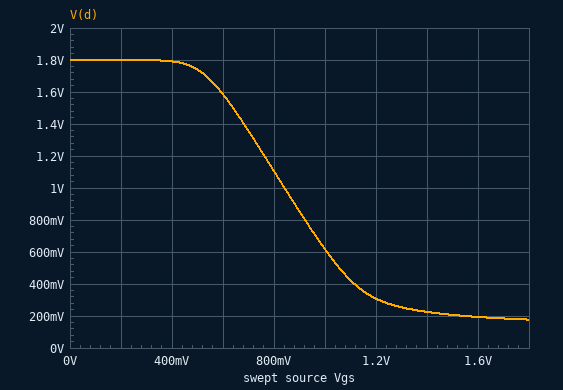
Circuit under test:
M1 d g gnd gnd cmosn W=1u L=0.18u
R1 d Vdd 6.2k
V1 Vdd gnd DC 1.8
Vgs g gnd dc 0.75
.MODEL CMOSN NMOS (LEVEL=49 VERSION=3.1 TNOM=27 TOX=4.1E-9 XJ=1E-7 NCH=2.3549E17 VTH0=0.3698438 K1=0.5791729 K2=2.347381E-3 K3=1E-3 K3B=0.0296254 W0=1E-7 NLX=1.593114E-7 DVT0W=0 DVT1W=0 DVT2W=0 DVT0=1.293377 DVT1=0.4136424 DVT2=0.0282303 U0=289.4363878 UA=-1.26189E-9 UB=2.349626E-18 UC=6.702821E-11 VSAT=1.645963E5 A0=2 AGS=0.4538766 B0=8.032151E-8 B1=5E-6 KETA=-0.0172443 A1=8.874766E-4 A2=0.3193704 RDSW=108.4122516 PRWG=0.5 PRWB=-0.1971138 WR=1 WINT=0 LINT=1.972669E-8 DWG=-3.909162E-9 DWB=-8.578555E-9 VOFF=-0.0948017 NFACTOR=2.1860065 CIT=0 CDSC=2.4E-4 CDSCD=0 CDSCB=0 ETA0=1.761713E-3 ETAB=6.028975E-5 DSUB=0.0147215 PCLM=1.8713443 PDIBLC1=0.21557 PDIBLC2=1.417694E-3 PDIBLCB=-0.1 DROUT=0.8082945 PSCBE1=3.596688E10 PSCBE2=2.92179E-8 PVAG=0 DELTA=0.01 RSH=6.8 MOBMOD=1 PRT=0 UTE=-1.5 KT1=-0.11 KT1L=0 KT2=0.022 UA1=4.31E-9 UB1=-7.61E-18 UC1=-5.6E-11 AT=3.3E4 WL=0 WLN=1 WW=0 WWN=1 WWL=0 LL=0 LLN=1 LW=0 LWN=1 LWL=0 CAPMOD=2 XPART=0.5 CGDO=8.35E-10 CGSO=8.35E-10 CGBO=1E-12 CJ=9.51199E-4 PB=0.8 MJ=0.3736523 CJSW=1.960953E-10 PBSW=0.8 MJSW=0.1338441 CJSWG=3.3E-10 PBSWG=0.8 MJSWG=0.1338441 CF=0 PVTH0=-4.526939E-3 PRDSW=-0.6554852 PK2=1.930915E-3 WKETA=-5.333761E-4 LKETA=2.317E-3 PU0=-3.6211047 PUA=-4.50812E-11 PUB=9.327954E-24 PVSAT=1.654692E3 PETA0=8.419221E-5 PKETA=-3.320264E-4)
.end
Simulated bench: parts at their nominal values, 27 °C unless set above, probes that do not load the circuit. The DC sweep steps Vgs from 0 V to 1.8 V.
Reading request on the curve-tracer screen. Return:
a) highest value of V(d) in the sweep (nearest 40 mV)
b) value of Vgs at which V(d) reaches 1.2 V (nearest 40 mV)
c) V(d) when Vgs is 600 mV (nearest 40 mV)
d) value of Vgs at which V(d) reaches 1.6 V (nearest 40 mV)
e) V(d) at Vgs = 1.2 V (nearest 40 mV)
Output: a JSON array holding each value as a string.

["1.80 V", "760 mV", "1.60 V", "600 mV", "320 mV"]
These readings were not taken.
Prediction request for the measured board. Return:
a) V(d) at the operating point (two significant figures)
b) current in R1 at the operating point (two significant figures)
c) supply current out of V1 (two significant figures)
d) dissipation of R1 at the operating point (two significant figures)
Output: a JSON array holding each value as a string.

["1.2 V", "92 µA", "92 µA", "52 µW"]
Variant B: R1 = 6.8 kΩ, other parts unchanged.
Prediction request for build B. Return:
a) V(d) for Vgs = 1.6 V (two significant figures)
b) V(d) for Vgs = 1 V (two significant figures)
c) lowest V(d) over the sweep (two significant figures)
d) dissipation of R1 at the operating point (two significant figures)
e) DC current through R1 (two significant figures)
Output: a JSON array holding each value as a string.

["180 mV", "530 mV", "160 mV", "56 µW", "91 µA"]
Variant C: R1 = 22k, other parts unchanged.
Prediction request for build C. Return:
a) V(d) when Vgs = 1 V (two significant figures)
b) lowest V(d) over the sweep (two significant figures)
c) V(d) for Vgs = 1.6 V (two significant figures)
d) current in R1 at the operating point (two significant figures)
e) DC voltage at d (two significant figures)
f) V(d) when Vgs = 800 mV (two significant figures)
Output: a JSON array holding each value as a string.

["94 mV", "49 mV", "53 mV", "69 µA", "280 mV", "180 mV"]
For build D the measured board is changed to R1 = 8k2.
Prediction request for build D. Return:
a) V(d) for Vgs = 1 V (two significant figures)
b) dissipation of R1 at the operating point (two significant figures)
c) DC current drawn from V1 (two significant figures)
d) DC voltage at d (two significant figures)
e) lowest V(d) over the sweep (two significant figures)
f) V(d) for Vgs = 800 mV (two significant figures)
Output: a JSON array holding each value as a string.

["370 mV", "65 µW", "89 µA", "1.1 V", "130 mV", "910 mV"]
